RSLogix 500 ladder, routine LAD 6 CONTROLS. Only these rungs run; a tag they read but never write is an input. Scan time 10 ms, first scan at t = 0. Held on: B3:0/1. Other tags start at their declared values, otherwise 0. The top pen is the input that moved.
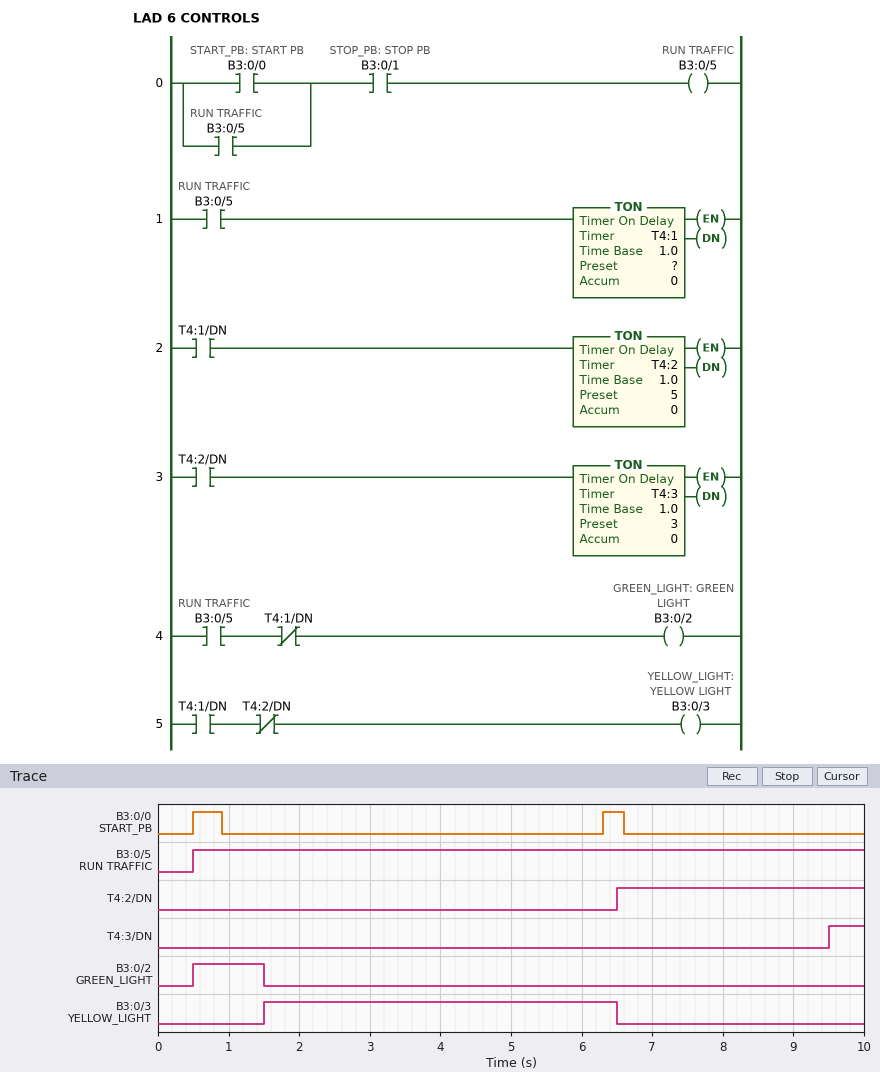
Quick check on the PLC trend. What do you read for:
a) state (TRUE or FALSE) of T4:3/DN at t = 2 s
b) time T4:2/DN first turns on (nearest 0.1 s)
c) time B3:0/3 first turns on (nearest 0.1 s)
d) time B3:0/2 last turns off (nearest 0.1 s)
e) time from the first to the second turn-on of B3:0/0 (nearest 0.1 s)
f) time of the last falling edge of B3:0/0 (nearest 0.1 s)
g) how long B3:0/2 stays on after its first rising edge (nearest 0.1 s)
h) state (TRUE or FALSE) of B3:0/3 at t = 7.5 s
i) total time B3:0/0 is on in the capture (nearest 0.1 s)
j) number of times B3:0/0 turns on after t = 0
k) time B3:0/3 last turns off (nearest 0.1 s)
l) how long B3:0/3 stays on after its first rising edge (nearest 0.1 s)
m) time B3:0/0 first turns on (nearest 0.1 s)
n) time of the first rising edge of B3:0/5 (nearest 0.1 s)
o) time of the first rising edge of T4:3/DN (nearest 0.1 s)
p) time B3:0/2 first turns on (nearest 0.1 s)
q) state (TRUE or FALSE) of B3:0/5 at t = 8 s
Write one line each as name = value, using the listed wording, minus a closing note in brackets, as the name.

state (TRUE or FALSE) of T4:3/DN at t = 2 s = FALSE
time T4:2/DN first turns on = 6.5 s
time B3:0/3 first turns on = 1.5 s
time B3:0/2 last turns off = 1.5 s
time from the first to the second turn-on of B3:0/0 = 5.8 s
time of the last falling edge of B3:0/0 = 6.6 s
how long B3:0/2 stays on after its first rising edge = 1.0 s
state (TRUE or FALSE) of B3:0/3 at t = 7.5 s = FALSE
total time B3:0/0 is on in the capture = 0.7 s
number of times B3:0/0 turns on after t = 0 = 2
time B3:0/3 last turns off = 6.5 s
how long B3:0/3 stays on after its first rising edge = 5.0 s
time B3:0/0 first turns on = 0.5 s
time of the first rising edge of B3:0/5 = 0.5 s
time of the first rising edge of T4:3/DN = 9.5 s
time B3:0/2 first turns on = 0.5 s
state (TRUE or FALSE) of B3:0/5 at t = 8 s = TRUE
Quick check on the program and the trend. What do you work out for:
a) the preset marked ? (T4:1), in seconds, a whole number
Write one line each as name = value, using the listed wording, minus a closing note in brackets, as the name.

the preset marked ? (T4:1), in seconds, a whole number = 1 s
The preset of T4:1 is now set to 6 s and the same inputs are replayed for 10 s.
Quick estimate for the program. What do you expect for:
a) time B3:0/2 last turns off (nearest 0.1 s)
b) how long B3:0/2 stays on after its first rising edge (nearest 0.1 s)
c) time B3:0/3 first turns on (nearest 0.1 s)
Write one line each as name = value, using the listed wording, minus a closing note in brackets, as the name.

time B3:0/2 last turns off = 6.5 s
how long B3:0/2 stays on after its first rising edge = 6.0 s
time B3:0/3 first turns on = 6.5 s
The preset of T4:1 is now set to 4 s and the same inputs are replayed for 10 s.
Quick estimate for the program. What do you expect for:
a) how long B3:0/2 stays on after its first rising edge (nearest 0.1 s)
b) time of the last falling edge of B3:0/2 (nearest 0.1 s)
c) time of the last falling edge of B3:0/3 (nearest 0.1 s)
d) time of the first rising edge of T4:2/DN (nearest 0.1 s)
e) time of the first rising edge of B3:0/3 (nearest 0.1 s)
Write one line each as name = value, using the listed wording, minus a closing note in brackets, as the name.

how long B3:0/2 stays on after its first rising edge = 4.0 s
time of the last falling edge of B3:0/2 = 4.5 s
time of the last falling edge of B3:0/3 = 9.5 s
time of the first rising edge of T4:2/DN = 9.5 s
time of the first rising edge of B3:0/3 = 4.5 s
